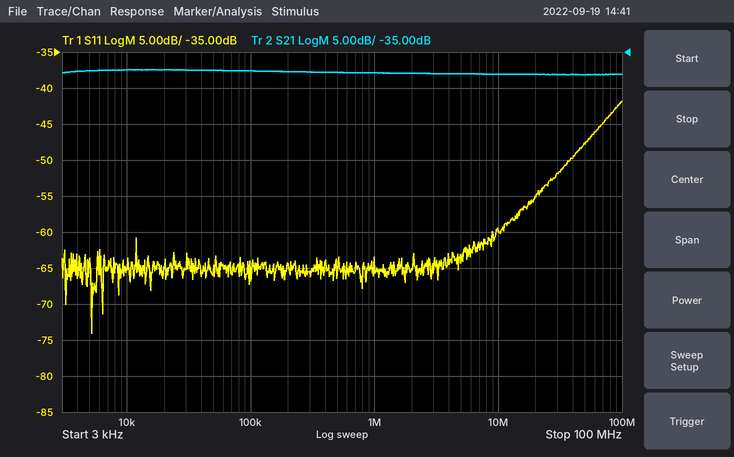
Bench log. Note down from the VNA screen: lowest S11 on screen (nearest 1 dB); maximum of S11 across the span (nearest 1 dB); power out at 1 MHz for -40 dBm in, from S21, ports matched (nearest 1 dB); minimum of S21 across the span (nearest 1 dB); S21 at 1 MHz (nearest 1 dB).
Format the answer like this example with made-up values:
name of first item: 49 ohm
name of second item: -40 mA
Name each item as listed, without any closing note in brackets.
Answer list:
lowest S11 on screen: -74 dB
maximum of S11 across the span: -42 dB
power out at 1 MHz for -40 dBm in, from S21, ports matched: -78 dBm
minimum of S21 across the span: -38 dB
S21 at 1 MHz: -38 dB
